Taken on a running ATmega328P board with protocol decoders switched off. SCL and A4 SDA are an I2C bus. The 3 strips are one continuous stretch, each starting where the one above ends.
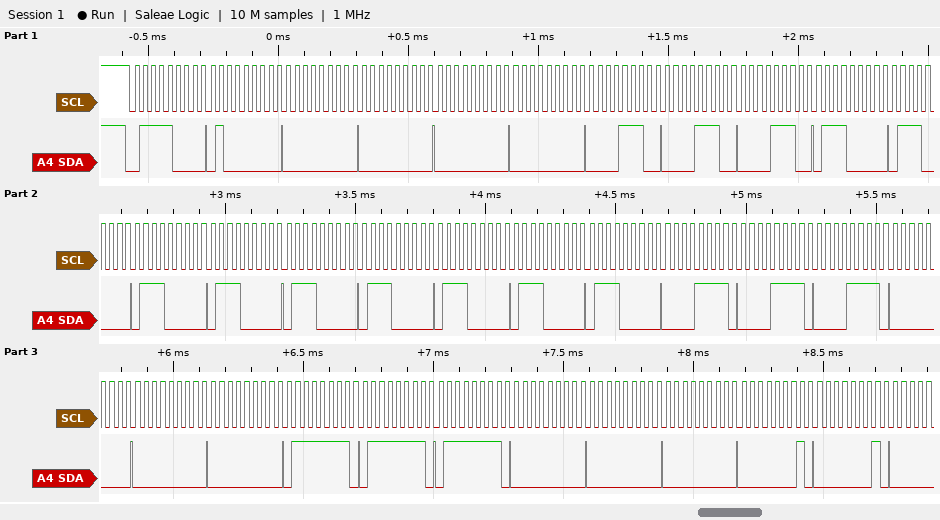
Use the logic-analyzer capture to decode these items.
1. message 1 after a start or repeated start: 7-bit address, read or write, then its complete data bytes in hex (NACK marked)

0x3C write: 40 00 00 00 00 0E 0E 0E 70 70 70 70 70 70 70 70 70 0F 0F 0F 00 00 00 7F 7F 7F 00 00 00 01 01
